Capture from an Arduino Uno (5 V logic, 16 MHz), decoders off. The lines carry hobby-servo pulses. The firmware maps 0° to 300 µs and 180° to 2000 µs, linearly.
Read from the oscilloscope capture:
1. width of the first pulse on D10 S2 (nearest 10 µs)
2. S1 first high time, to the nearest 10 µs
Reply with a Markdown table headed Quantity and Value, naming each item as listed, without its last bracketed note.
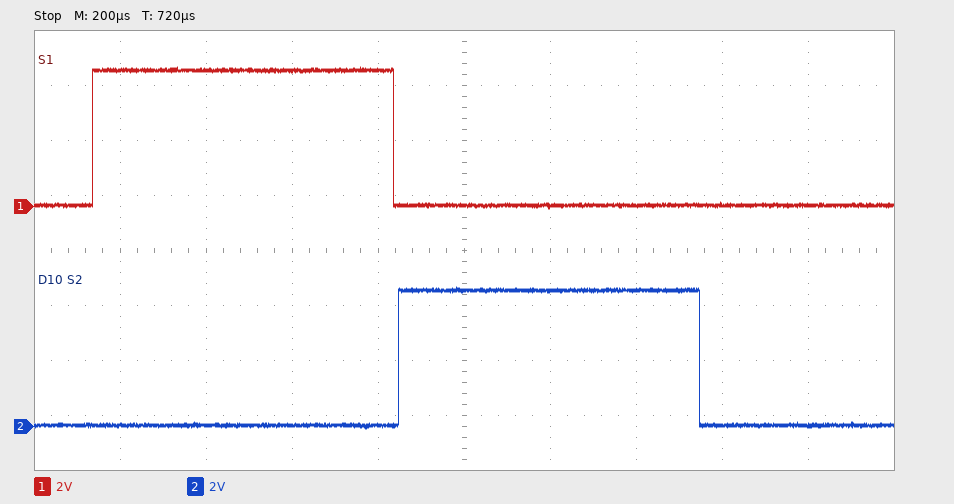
| Quantity | Value |
|---|---|
| width of the first pulse on D10 S2 | 700 µs |
| S1 first high time, to the nearest 10 µs | 700 µs |
